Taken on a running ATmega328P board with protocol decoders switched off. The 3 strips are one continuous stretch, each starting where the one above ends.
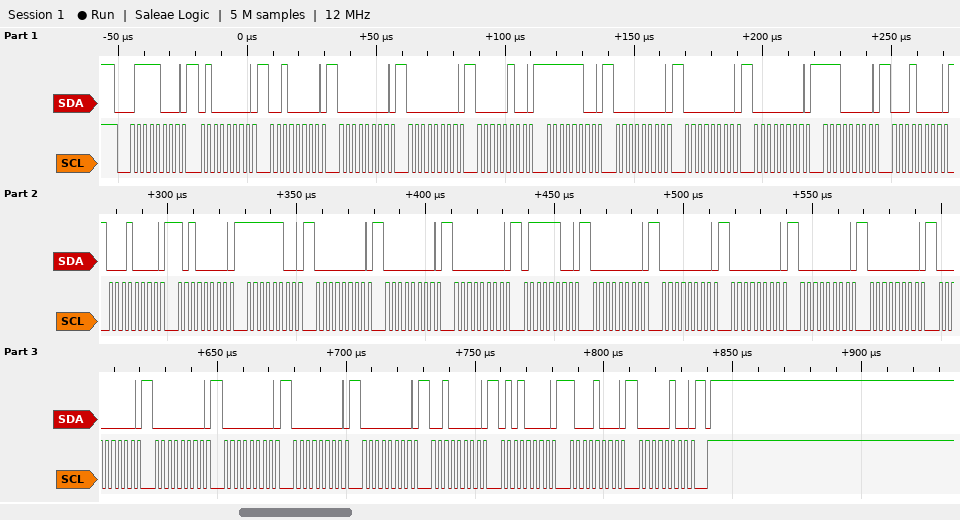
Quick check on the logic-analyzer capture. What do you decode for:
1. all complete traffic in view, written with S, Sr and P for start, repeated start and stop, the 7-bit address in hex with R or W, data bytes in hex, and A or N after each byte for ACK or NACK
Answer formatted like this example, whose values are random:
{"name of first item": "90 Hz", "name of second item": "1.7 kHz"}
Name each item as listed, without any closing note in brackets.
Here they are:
{"all complete traffic in view, written with S, Sr and P for start, repeated start and stop, the 7-bit address in hex with R or W, data bytes in hex, and A or N after each byte for ACK or NACK": "S 3CW A 40 A 20 A 00 A 00 A 04 A FC A 00 A 00 A 00 A E0 A 10 A 10 A A0 A FC A 00 A 00 A 00 A 7C A 00 A 00 A 00 A 00 A 00 A 00 A 00 A 00 A 00 A 00 A 20 A 50 A 88 A 04 A P"}
